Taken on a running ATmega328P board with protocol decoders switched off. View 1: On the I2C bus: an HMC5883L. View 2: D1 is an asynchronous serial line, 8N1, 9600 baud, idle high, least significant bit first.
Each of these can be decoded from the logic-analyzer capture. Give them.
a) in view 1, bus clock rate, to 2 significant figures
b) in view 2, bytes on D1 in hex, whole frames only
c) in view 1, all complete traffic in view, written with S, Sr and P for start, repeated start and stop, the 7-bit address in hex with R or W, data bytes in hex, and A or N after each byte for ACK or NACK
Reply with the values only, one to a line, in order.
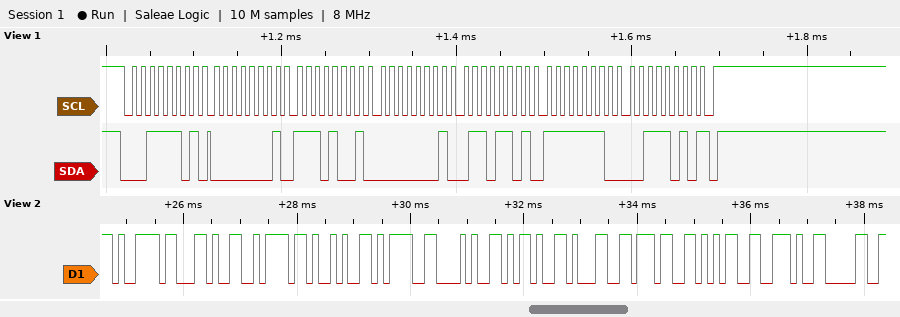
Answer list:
100 kHz
79 2C 7A 29 3D 28 2D 31 37 35 2E 30
S 1ER A 01 A E9 A 01 A 6D A FE A 3A N P
